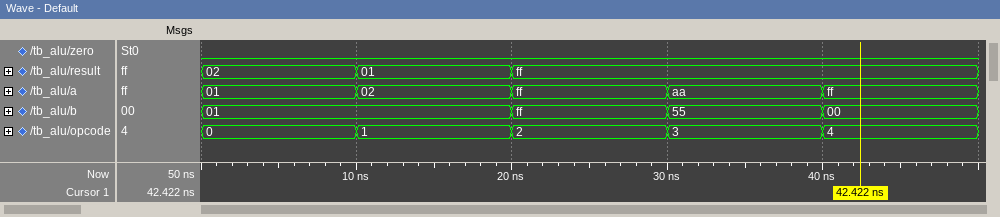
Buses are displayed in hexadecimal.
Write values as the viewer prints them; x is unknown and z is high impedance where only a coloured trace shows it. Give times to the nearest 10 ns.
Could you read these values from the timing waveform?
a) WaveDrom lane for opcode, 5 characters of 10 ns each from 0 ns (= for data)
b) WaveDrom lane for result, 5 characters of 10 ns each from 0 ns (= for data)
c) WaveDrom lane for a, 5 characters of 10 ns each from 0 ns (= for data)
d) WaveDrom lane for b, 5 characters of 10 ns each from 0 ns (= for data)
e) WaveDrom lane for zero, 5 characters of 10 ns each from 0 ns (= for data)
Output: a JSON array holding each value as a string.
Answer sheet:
["{name: 'opcode', wave: '=====', data: '0 1 2 3 4'}", "{name: 'result', wave: '===..', data: '02 01 ff'}", "{name: 'a', wave: '=====', data: '01 02 ff aa ff'}", "{name: 'b', wave: '=.===', data: '01 ff 55 00'}", "{name: 'zero', wave: '0....'}"]
